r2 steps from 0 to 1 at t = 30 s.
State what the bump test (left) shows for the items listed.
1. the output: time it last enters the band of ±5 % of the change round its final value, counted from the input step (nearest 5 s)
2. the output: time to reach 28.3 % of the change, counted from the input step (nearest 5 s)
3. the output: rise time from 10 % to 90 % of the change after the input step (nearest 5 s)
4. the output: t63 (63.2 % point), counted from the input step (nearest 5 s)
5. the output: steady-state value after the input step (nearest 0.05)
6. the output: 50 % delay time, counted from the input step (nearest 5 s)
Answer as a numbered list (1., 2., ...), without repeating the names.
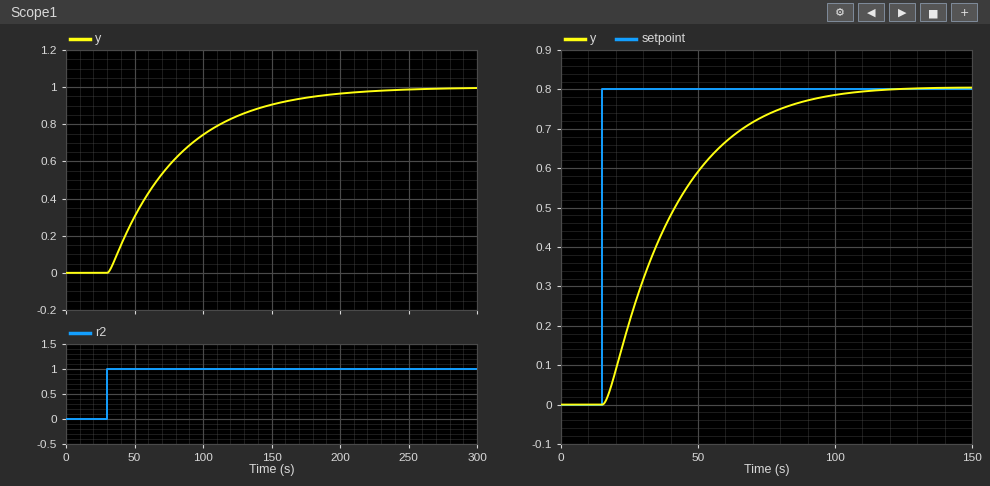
1. 150 s
2. 20 s
3. 110 s
4. 50 s
5. 1.00
6. 35 s
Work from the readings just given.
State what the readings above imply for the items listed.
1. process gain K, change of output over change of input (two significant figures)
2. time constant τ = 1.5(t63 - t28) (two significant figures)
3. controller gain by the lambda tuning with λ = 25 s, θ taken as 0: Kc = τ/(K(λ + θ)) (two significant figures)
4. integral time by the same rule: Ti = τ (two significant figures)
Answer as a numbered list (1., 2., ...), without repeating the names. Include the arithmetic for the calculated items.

1. (1 - 0) / 1 = 1.0
2. 1.5 × (50 - 20) = 45 s
3. 45 / (1 × (25 + 0)) = 1.8
4. 45 s
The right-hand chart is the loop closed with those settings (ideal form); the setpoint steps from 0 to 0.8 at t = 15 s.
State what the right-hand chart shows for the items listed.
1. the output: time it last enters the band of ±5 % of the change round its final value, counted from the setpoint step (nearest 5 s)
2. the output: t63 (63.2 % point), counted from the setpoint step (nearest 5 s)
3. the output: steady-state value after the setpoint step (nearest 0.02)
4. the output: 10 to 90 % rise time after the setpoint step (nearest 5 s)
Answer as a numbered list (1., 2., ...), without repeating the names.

1. 70 s
2. 25 s
3. 0.80
4. 50 s
